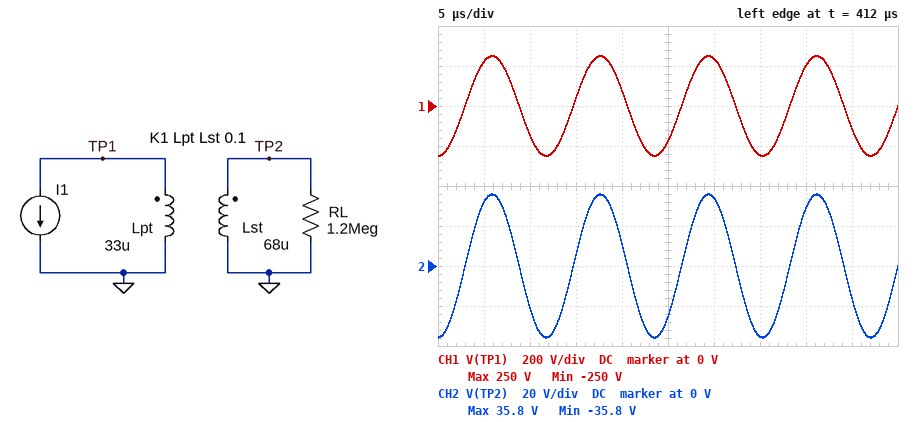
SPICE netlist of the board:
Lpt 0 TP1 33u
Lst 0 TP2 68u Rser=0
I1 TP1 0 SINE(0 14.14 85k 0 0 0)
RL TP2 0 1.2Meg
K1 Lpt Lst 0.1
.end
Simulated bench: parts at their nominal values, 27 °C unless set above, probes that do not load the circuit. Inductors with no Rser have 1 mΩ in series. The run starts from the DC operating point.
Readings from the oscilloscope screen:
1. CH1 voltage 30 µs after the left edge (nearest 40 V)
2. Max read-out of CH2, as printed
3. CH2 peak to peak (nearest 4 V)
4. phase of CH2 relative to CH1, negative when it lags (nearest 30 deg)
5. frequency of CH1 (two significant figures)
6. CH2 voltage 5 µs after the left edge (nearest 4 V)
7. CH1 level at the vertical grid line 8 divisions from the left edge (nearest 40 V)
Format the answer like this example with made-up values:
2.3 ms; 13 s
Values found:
240 V; 35.8 V; 72 V; 0 deg; 85 kHz; 32 V; 200 V
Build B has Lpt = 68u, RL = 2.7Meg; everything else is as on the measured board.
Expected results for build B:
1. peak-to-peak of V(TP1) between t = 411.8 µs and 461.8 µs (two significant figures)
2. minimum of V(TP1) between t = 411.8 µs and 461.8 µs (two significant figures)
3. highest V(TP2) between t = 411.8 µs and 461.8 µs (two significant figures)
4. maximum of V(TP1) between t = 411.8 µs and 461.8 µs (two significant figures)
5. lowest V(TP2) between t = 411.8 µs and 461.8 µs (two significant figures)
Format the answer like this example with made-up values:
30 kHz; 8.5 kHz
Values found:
1.0 kV; -510 V; 51 V; 510 V; -51 V
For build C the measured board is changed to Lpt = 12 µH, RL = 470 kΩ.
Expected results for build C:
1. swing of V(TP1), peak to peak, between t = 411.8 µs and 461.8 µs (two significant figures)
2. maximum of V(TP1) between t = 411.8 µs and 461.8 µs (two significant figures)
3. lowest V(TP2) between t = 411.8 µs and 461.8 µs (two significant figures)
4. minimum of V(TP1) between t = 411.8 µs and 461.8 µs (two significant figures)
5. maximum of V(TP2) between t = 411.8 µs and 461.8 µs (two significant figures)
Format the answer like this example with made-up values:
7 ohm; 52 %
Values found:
180 V; 91 V; -22 V; -91 V; 22 V
